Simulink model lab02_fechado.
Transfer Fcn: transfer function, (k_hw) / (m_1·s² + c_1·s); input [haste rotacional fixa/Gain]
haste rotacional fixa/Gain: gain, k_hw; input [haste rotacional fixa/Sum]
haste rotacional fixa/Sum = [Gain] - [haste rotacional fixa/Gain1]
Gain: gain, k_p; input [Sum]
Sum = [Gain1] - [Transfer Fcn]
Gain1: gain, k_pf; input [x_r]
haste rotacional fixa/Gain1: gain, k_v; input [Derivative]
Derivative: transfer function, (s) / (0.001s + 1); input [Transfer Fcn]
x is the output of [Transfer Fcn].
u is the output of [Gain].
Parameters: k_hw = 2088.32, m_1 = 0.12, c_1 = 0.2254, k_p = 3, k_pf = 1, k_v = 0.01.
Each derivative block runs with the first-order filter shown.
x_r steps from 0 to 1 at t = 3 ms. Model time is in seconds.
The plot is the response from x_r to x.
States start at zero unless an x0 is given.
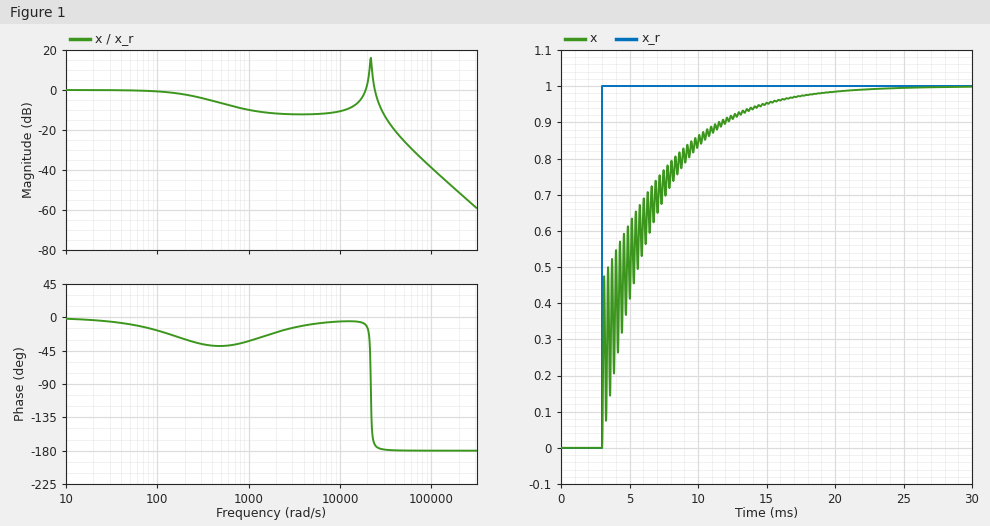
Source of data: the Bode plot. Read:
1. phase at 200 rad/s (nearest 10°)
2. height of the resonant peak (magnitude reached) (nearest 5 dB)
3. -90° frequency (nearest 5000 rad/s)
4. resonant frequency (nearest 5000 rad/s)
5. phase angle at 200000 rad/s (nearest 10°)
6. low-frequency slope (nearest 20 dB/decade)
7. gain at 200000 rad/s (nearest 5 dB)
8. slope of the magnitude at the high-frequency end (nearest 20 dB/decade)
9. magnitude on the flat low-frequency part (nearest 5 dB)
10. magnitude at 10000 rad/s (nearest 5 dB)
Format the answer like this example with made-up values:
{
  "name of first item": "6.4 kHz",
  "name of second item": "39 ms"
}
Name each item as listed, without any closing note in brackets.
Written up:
{
  "phase at 200 rad/s": "-30°",
  "height of the resonant peak (magnitude reached)": "15 dB",
  "-90° frequency": "20000 rad/s",
  "resonant frequency": "20000 rad/s",
  "phase angle at 200000 rad/s": "-180°",
  "low-frequency slope": "0 dB/decade",
  "gain at 200000 rad/s": "-50 dB",
  "slope of the magnitude at the high-frequency end": "-40 dB/decade",
  "magnitude on the flat low-frequency part": "0 dB",
  "magnitude at 10000 rad/s": "-10 dB"
}
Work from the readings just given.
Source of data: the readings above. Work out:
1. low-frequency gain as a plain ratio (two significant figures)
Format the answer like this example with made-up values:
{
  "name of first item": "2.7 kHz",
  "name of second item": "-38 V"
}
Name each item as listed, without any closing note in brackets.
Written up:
{
  "low-frequency gain as a plain ratio": "1.0"
}
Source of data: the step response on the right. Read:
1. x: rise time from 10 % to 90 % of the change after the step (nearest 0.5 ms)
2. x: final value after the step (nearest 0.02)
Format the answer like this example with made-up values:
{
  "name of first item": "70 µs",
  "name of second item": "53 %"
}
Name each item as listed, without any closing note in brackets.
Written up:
{
  "x: rise time from 10 % to 90 % of the change after the step": "8.5 ms",
  "x: final value after the step": "1.00"
}
